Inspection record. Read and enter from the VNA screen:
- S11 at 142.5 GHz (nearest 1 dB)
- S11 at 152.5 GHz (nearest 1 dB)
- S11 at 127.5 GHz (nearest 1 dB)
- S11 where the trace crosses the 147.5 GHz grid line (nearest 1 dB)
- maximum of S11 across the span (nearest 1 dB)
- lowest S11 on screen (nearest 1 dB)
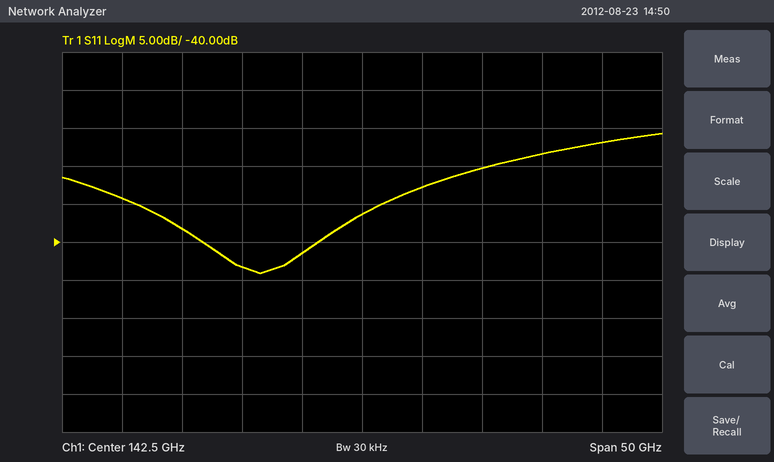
-36 dB
-30 dB
-38 dB
-33 dB
-26 dB
-44 dB
